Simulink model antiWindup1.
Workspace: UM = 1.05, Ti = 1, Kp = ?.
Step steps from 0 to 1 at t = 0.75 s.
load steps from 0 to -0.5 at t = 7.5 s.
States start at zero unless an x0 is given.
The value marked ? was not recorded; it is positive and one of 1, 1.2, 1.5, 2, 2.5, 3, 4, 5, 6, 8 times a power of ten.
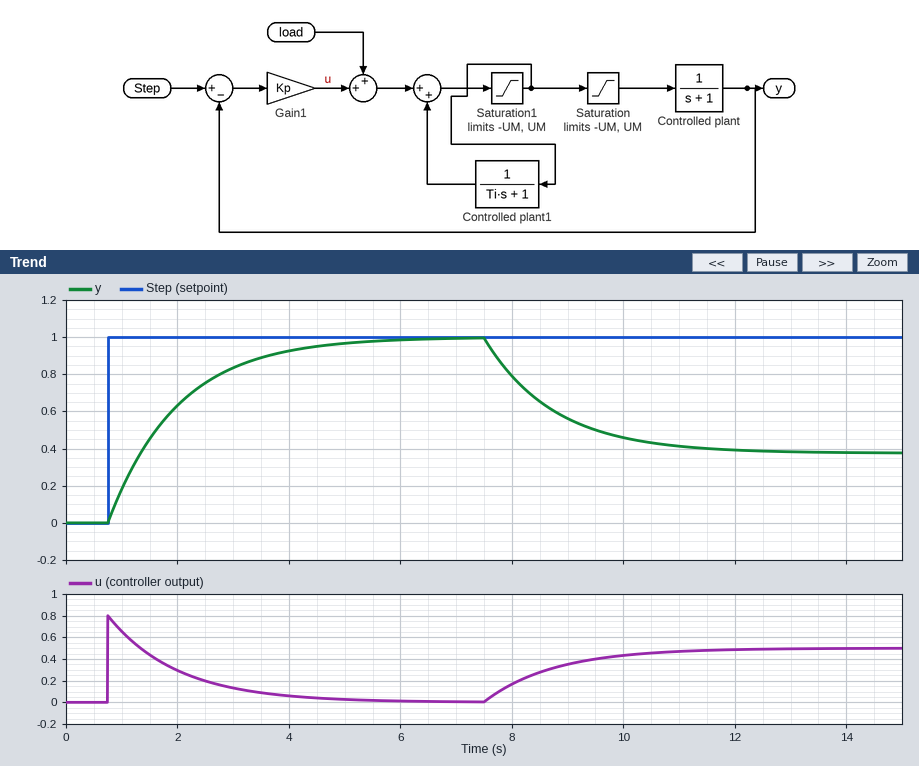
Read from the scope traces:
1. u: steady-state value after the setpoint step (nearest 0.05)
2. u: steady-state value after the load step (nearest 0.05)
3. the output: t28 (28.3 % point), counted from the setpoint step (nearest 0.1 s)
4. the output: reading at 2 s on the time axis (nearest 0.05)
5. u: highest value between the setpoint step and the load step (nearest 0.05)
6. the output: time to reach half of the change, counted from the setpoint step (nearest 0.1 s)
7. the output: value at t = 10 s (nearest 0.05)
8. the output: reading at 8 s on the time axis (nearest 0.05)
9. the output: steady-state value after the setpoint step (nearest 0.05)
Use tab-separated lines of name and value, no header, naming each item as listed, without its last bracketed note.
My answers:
u: steady-state value after the setpoint step	0.00
u: steady-state value after the load step	0.50
the output: t28 (28.3 % point), counted from the setpoint step	0.4 s
the output: reading at 2 s on the time axis	0.65
u: highest value between the setpoint step and the load step	0.80
the output: time to reach half of the change, counted from the setpoint step	0.9 s
the output: value at t = 10 s	0.45
the output: reading at 8 s on the time axis	0.80
the output: steady-state value after the setpoint step	1.00
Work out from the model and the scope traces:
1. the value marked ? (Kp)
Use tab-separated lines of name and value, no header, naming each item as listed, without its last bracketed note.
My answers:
the value marked ?	0.8
